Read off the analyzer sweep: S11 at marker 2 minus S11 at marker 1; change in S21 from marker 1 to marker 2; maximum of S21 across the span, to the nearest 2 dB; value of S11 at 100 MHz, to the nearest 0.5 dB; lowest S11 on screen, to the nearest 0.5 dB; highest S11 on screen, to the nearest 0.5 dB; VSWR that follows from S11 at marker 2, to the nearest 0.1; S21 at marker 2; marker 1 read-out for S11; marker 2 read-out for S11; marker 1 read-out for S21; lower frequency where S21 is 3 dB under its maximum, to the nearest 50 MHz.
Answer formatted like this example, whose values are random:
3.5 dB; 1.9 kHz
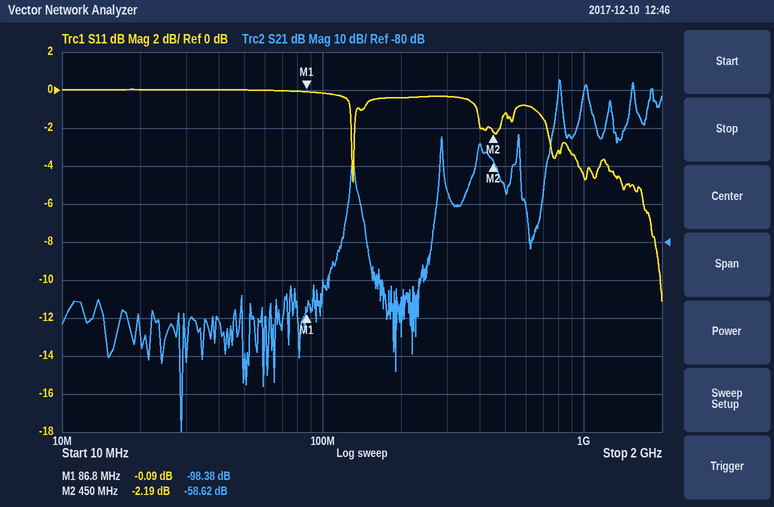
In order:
-2.10 dB; 39.76 dB; -38 dB; 0.0 dB; -11.0 dB; 0.0 dB; 8.0; -58.62 dB; -0.09 dB; -2.19 dB; -98.38 dB; 800 MHz
